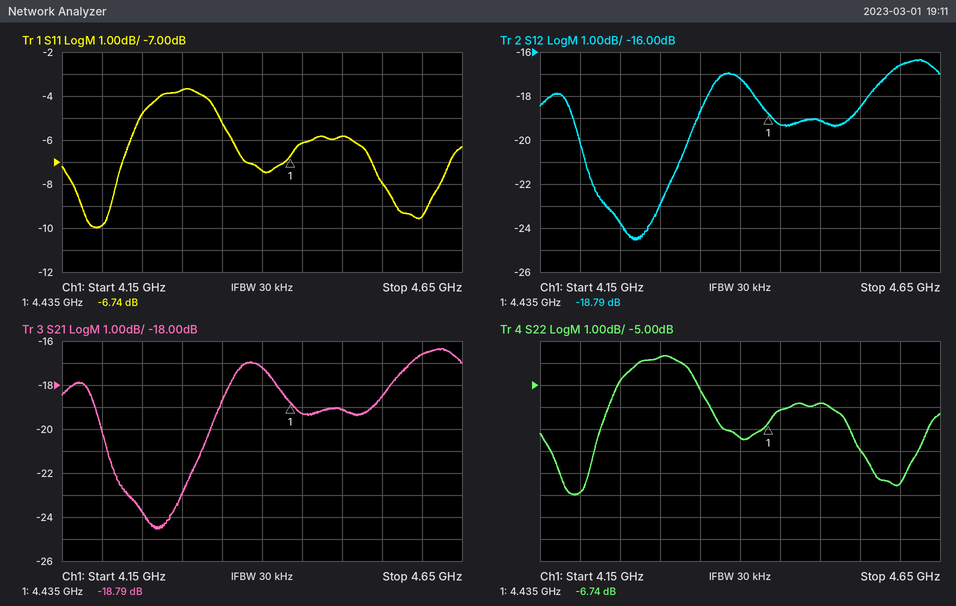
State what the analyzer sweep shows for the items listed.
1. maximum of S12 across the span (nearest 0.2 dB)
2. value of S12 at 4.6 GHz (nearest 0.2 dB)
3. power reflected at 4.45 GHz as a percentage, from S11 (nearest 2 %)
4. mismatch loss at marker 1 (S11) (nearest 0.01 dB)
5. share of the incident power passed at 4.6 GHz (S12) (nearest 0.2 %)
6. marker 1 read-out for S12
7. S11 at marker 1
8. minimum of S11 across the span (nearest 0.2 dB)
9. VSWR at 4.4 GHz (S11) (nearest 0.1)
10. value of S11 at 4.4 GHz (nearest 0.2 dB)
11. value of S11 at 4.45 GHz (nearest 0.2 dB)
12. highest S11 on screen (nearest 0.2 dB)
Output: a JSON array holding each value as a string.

["-16.4 dB", "-16.6 dB", "24 %", "1.03 dB", "2.2 %", "-18.79 dB", "-6.74 dB", "-10.0 dB", "2.5", "-7.4 dB", "-6.2 dB", "-3.6 dB"]
